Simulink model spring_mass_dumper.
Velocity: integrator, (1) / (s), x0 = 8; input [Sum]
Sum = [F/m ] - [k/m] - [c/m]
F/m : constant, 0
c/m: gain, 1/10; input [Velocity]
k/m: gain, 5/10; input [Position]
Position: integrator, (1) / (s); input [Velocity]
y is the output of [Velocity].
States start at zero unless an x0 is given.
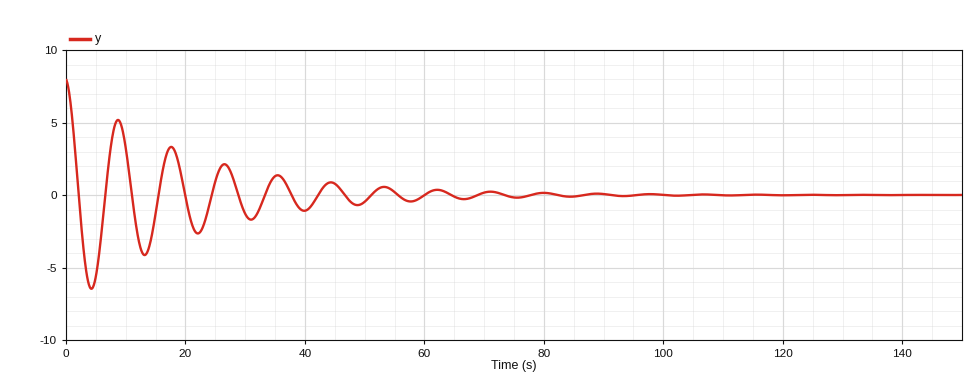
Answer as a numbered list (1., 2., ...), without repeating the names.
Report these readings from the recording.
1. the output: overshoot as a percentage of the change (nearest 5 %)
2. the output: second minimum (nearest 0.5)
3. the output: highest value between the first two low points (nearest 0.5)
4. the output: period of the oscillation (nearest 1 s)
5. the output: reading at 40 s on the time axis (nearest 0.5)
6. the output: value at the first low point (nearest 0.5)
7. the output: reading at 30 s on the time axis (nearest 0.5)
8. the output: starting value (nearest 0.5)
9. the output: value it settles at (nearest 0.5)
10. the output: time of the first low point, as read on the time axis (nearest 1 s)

1. 80 %
2. -4.0
3. 5.0
4. 9 s
5. -1.0
6. -6.5
7. -1.5
8. 8.0
9. 0.0
10. 4 s
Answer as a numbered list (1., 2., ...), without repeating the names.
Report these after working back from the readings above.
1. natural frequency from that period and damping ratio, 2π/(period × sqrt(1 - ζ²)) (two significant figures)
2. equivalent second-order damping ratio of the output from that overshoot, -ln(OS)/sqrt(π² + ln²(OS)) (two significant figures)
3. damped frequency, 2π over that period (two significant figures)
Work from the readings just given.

1. 0.70 rad/s
2. 0.071
3. 0.70 rad/s
